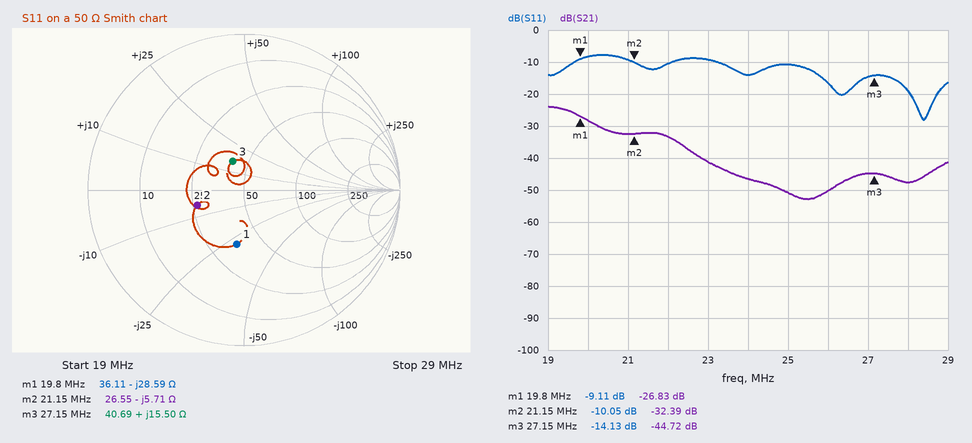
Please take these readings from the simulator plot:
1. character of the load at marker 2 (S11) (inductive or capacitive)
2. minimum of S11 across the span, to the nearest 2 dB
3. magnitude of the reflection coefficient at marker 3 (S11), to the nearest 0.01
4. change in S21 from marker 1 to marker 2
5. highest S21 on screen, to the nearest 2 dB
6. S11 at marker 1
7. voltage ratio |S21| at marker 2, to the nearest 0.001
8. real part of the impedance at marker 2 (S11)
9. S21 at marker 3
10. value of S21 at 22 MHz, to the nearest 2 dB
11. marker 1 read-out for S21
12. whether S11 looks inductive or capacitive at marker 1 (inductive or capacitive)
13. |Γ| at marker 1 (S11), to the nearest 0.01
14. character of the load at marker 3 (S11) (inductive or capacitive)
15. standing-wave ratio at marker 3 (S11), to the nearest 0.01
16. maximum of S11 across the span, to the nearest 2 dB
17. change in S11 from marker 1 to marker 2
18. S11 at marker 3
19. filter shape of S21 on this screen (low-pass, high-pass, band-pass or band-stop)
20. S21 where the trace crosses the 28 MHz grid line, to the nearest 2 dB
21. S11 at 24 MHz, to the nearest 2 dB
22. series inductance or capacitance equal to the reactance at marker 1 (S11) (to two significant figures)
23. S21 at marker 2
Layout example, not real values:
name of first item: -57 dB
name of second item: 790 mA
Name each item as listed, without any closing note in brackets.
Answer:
character of the load at marker 2 (S11): capacitive
minimum of S11 across the span, to the nearest 2 dB: -28 dB
magnitude of the reflection coefficient at marker 3 (S11), to the nearest 0.01: 0.20
change in S21 from marker 1 to marker 2: -5.56 dB
highest S21 on screen, to the nearest 2 dB: -24 dB
S11 at marker 1: -9.11 dB
voltage ratio |S21| at marker 2, to the nearest 0.001: 0.024
real part of the impedance at marker 2: 26.55 Ω
S21 at marker 3: -44.72 dB
value of S21 at 22 MHz, to the nearest 2 dB: -34 dB
marker 1 read-out for S21: -26.83 dB
whether S11 looks inductive or capacitive at marker 1: capacitive
|Γ| at marker 1 (S11), to the nearest 0.01: 0.35
character of the load at marker 3 (S11): inductive
standing-wave ratio at marker 3 (S11), to the nearest 0.01: 1.49
maximum of S11 across the span, to the nearest 2 dB: -8 dB
change in S11 from marker 1 to marker 2: -0.94 dB
S11 at marker 3: -14.13 dB
filter shape of S21 on this screen: low-pass
S21 where the trace crosses the 28 MHz grid line, to the nearest 2 dB: -48 dB
S11 at 24 MHz, to the nearest 2 dB: -14 dB
series inductance or capacitance equal to the reactance at marker 1 (S11): 280 pF
S21 at marker 2: -32.39 dB
